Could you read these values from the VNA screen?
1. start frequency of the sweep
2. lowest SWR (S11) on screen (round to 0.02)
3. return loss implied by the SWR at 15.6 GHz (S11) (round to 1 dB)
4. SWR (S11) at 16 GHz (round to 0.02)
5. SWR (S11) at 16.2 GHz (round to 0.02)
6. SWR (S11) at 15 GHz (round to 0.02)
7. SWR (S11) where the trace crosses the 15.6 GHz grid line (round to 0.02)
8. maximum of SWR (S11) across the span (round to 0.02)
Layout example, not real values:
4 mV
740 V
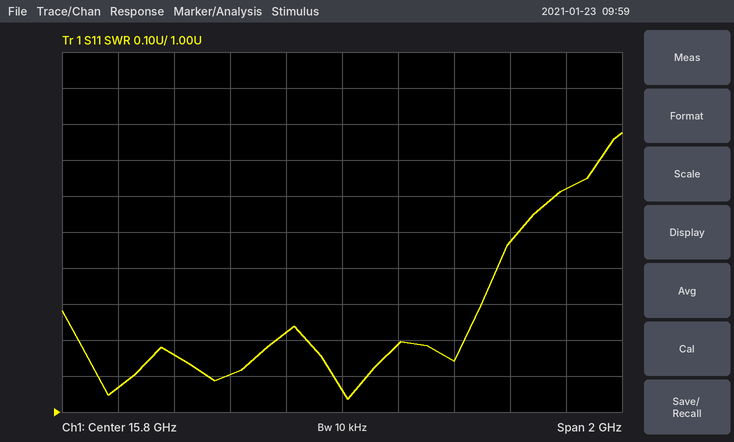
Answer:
14.8 GHz
1.04
20 dB
1.18
1.14
1.06
1.22
1.78
